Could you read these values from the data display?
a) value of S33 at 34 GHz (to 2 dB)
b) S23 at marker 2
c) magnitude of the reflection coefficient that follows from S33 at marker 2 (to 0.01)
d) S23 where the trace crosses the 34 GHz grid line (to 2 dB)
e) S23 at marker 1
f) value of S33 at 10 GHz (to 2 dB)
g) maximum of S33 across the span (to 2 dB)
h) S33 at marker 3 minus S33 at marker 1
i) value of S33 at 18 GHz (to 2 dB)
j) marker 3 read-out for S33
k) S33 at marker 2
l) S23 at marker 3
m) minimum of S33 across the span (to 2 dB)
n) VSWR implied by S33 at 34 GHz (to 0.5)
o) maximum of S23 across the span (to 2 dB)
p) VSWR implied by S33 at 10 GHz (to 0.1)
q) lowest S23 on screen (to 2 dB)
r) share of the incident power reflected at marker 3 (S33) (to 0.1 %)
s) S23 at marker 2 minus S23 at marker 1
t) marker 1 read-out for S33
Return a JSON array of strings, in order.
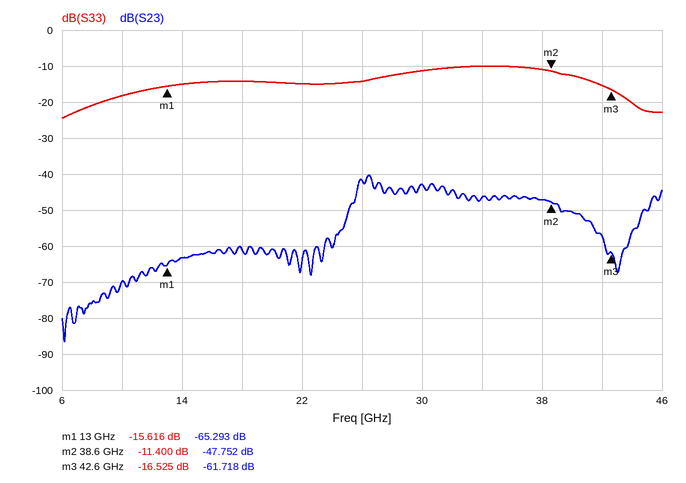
["-10 dB", "-47.752 dB", "0.27", "-46 dB", "-65.293 dB", "-18 dB", "-10 dB", "-0.909 dB", "-14 dB", "-16.525 dB", "-11.400 dB", "-61.718 dB", "-24 dB", "2.0", "-40 dB", "1.3", "-86 dB", "2.2 %", "17.541 dB", "-15.616 dB"]
